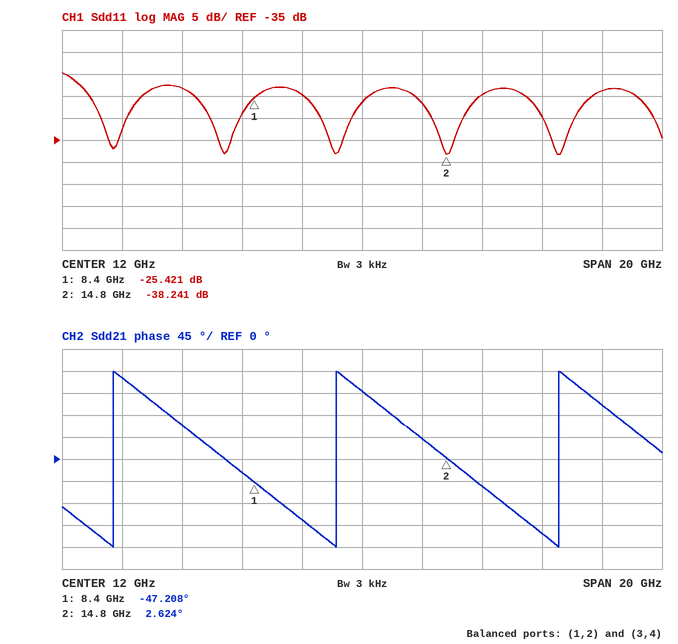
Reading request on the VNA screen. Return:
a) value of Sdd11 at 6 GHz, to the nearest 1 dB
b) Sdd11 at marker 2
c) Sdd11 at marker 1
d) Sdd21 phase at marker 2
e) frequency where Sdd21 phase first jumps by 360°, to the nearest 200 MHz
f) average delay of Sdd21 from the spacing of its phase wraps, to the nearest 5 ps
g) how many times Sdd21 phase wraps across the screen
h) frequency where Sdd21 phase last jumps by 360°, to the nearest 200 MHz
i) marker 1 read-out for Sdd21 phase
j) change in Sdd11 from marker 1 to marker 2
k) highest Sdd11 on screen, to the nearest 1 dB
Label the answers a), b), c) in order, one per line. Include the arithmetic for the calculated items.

a) -23 dB
b) -38.241 dB
c) -25.421 dB
d) 2.624°
e) 3.8 GHz
f) 2 cycles / (18.6 GHz − 3.8 GHz) ≈ 135 ps
g) 3
h) 18.6 GHz
i) -47.208°
j) -38.241 − (-25.421) = -12.820 dB
k) -20 dB
